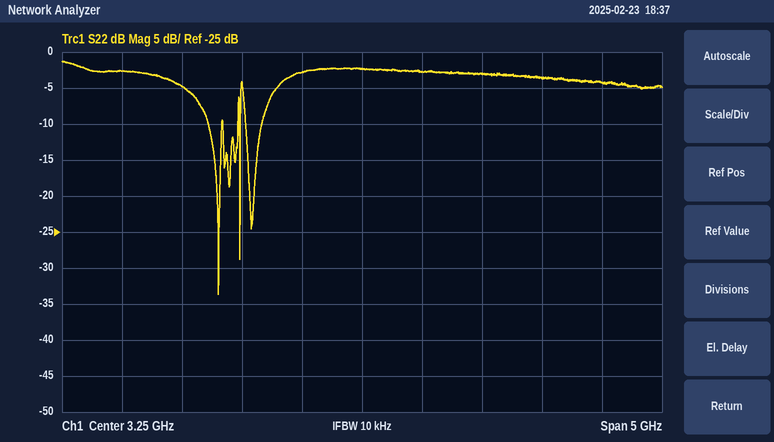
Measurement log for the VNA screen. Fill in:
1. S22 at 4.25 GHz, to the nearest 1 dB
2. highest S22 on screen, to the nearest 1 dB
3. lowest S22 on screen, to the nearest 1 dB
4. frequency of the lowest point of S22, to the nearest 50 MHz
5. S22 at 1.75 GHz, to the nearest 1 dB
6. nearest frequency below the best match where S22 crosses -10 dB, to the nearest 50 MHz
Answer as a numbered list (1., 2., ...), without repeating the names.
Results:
1. -3 dB
2. -1 dB
3. -34 dB
4. 2.05 GHz
5. -5 dB
6. 1.95 GHz
